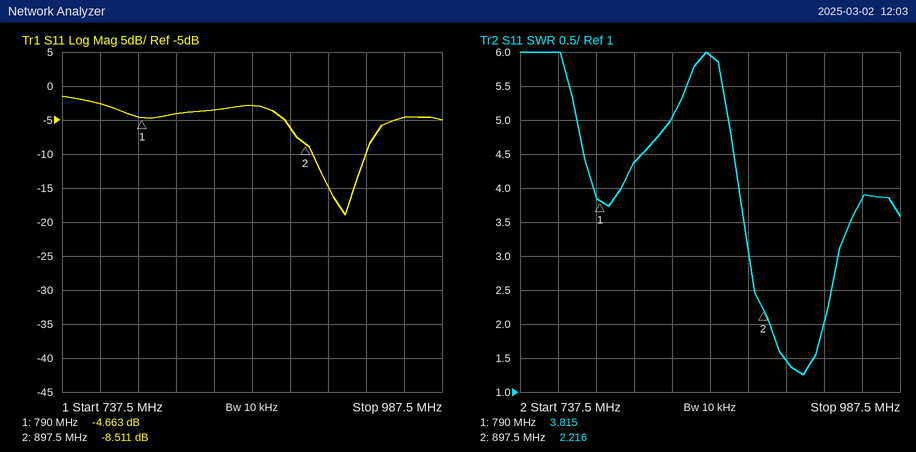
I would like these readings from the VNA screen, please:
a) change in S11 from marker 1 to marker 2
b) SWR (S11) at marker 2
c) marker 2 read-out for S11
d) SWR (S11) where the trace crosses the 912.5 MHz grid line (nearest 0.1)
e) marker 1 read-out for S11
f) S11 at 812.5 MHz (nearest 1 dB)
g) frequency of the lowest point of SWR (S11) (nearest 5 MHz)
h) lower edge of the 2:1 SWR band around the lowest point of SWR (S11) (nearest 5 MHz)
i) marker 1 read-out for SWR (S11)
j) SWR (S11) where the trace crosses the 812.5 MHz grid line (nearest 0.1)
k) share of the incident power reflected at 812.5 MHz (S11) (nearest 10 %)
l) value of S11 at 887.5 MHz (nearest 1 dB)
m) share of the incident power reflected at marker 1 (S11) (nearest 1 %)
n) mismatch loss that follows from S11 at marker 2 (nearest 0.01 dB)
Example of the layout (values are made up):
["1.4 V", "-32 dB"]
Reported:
["-3.848 dB", "2.216", "-8.511 dB", "1.5", "-4.663 dB", "-4 dB", "925 MHz", "900 MHz", "3.815", "4.4", "40 %", "-6 dB", "34 %", "0.66 dB"]
